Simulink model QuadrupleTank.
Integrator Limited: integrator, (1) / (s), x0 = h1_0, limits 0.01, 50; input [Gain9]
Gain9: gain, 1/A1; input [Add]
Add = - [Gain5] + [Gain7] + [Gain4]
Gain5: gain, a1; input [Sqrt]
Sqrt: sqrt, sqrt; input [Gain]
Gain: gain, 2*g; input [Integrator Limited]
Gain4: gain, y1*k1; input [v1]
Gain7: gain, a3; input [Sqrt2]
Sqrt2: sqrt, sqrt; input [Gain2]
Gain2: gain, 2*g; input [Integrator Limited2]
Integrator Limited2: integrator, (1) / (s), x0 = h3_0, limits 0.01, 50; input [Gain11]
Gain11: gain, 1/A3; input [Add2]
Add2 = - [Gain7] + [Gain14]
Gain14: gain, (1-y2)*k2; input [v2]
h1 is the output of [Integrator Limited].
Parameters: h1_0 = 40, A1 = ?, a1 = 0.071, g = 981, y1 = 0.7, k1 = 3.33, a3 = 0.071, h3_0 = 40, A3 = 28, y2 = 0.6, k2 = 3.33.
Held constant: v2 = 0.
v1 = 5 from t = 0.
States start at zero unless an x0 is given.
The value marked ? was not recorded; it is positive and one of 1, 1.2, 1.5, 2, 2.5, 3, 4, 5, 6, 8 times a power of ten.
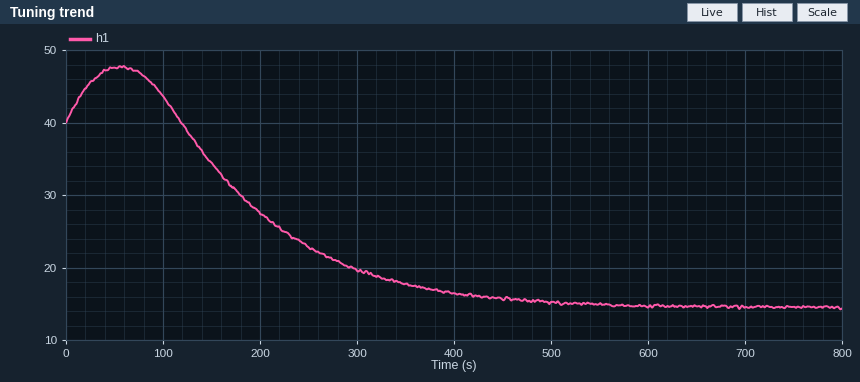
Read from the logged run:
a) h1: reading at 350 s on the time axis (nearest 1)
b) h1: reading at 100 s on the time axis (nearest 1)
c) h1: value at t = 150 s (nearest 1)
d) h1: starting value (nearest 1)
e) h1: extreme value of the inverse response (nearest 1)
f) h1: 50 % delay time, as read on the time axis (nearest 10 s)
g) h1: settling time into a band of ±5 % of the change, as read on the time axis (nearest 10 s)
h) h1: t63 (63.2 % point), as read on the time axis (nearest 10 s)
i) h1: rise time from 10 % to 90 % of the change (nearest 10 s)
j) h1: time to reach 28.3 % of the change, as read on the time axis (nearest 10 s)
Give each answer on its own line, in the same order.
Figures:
18
44
34
40
48
200 s
440 s
240 s
240 s
160 s
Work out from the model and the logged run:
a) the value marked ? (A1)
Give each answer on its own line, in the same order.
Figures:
40
